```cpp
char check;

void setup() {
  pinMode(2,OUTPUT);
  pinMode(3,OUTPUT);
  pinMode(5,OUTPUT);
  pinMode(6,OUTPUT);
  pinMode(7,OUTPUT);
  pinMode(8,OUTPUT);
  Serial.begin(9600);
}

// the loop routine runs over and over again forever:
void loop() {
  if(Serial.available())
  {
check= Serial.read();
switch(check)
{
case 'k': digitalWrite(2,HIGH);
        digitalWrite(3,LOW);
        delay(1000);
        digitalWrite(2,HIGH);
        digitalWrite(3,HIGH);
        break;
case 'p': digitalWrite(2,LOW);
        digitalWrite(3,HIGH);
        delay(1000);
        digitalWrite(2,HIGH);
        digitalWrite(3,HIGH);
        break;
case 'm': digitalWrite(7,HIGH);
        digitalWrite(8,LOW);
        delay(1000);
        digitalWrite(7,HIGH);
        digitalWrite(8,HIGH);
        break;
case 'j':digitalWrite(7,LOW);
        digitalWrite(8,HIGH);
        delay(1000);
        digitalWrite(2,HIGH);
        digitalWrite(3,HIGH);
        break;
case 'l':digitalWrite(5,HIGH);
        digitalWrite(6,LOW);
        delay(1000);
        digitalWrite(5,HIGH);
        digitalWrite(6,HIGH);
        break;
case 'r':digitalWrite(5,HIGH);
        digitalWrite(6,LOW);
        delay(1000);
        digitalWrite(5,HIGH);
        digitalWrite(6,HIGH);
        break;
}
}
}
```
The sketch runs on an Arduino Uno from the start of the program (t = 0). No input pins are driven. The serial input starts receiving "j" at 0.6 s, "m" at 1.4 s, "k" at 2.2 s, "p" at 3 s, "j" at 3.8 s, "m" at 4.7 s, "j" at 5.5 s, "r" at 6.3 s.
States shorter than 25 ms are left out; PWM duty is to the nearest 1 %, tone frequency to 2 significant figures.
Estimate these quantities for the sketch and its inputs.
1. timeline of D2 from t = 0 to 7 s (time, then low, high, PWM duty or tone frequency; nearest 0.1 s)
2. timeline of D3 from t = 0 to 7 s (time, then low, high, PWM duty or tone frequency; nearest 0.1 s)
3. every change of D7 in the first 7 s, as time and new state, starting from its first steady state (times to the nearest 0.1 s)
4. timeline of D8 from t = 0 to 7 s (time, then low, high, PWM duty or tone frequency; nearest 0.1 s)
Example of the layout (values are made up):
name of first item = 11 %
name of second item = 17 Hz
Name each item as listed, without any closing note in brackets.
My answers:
timeline of D2 from t = 0 to 7 s = 0 s low; 1.6 s high; 3.6 s low; 4.6 s high
timeline of D3 from t = 0 to 7 s = 0 s low; 1.6 s high; 2.6 s low; 3.6 s high
every change of D7 in the first 7 s, as time and new state, starting from its first steady state = 0 s low; 1.6 s high; 4.6 s low; 5.6 s high; 6.6 s low
timeline of D8 from t = 0 to 7 s = 0 s low; 0.6 s high; 1.6 s low; 2.6 s high; 5.6 s low; 6.6 s high
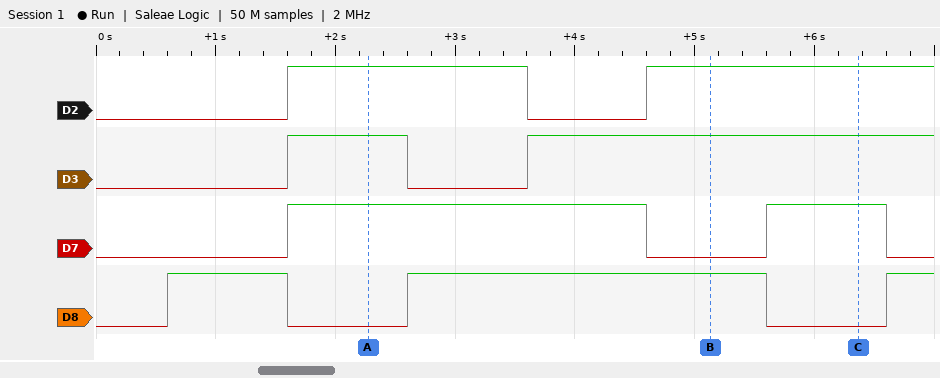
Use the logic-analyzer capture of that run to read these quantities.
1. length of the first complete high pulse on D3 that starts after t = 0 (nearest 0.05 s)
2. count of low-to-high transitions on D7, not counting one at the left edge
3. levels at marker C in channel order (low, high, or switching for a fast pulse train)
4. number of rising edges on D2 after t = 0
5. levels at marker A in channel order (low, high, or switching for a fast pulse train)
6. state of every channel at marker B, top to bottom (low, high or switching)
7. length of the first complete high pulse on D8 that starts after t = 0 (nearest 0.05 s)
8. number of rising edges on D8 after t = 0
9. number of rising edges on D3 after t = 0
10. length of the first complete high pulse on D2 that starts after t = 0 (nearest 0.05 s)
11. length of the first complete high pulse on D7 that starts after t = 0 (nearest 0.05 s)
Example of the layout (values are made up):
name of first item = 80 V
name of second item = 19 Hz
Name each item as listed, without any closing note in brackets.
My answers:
length of the first complete high pulse on D3 that starts after t = 0 = 1.00 s
count of low-to-high transitions on D7, not counting one at the left edge = 2
levels at marker C in channel order = D2 high, D3 high, D7 high, D8 low
number of rising edges on D2 after t = 0 = 2
levels at marker A in channel order = D2 high, D3 high, D7 high, D8 low
state of every channel at marker B, top to bottom = D2 high, D3 high, D7 low, D8 high
length of the first complete high pulse on D8 that starts after t = 0 = 1.00 s
number of rising edges on D8 after t = 0 = 3
number of rising edges on D3 after t = 0 = 2
length of the first complete high pulse on D2 that starts after t = 0 = 2.00 s
length of the first complete high pulse on D7 that starts after t = 0 = 3.00 s
